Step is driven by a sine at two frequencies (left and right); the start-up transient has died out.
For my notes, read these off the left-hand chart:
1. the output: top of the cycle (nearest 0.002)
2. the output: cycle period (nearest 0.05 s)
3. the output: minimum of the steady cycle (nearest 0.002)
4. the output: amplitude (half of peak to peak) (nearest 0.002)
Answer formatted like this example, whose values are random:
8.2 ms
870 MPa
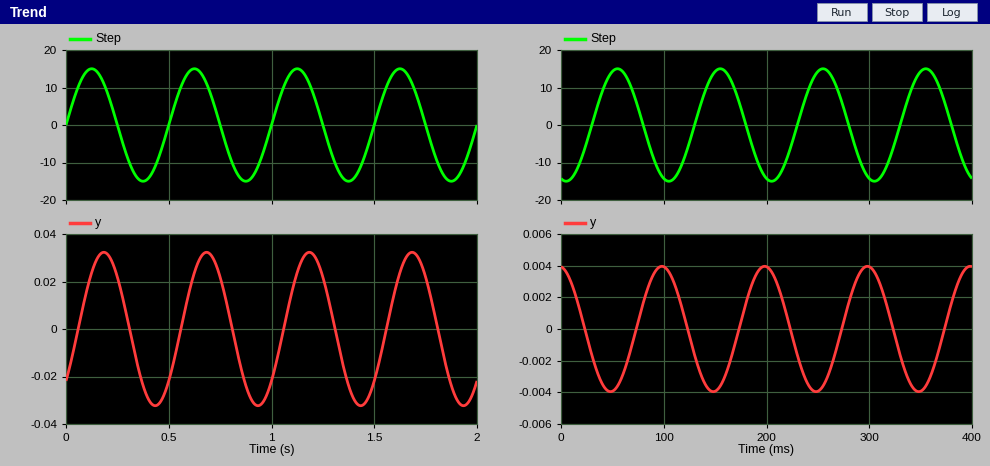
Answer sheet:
0.032
0.50 s
-0.032
0.032
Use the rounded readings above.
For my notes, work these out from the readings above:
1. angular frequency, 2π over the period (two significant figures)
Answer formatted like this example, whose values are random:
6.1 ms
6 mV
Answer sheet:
13 rad/s
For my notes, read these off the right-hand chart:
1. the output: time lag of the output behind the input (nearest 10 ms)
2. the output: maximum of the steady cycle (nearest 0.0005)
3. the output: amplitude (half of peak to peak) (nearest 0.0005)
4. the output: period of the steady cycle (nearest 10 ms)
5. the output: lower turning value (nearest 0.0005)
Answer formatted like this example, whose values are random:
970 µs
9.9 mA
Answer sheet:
40 ms
0.0040
0.0040
100 ms
-0.0040
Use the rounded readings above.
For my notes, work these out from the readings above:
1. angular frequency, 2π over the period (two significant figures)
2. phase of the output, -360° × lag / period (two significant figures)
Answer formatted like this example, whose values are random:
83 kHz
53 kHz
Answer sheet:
0.063 rad/ms
-140°
